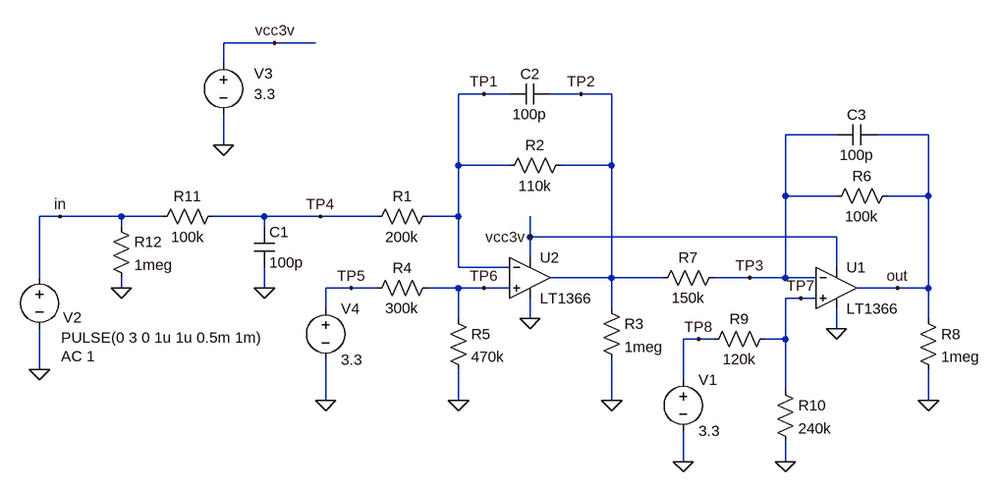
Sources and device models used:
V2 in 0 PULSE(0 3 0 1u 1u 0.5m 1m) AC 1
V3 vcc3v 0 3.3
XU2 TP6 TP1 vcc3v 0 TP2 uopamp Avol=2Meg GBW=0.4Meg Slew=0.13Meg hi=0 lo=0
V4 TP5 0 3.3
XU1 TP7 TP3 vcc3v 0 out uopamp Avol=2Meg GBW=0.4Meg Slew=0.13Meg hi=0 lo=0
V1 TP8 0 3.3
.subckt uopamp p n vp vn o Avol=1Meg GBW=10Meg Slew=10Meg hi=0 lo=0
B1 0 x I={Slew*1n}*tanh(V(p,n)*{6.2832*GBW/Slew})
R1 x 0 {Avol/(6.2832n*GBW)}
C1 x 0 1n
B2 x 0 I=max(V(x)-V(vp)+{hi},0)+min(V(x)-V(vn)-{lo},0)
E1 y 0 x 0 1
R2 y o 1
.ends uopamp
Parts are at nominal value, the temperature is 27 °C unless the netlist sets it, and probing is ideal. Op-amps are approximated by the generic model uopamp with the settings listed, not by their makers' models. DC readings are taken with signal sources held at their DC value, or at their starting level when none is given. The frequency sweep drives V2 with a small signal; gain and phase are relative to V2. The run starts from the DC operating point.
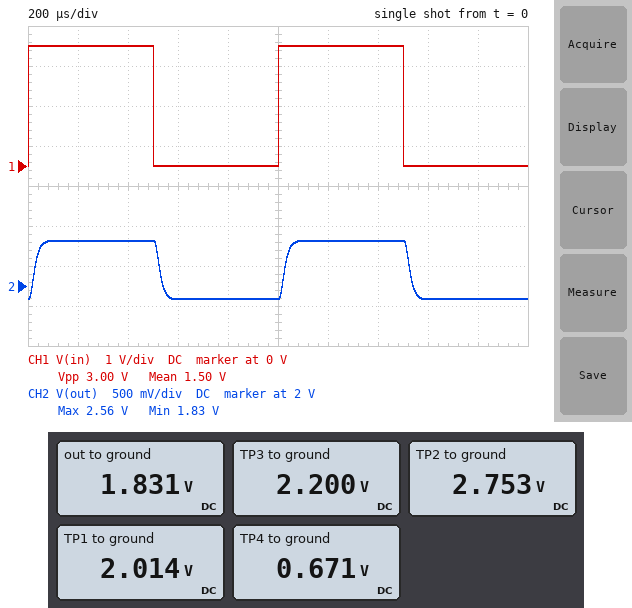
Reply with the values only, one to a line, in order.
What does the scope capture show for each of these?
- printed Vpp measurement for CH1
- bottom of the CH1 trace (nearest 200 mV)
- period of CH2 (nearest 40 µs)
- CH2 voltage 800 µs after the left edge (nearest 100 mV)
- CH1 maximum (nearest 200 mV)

3.00 V
0 V
1.00 ms
1.8 V
3.0 V
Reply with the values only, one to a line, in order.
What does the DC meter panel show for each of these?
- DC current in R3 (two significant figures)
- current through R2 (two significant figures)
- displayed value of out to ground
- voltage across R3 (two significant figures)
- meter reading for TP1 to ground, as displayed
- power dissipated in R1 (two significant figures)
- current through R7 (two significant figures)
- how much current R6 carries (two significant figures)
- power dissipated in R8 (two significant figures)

2.8 µA
6.7 µA
1.831 V
2.8 V
2.014 V
9.0 µW
3.7 µA
3.7 µA
3.4 µW
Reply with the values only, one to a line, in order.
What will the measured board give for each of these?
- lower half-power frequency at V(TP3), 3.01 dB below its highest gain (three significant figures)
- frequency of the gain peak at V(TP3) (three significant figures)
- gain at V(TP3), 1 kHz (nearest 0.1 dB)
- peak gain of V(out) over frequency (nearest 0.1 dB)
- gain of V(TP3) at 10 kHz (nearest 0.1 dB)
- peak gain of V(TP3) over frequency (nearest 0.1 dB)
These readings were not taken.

5.29 kHz
12.1 kHz
-64.3 dB
-12.2 dB
-48.2 dB
-48.0 dB
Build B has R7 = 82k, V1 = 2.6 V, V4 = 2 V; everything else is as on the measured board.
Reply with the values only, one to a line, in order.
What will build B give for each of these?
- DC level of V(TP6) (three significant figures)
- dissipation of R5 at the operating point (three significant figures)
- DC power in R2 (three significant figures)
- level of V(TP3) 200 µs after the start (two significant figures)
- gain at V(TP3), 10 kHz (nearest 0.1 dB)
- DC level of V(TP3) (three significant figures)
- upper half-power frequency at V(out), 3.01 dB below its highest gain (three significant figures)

1.22 V
3.17 µW
1.82 µW
1.7 V
-43.0 dB
1.73 V
8.48 kHz
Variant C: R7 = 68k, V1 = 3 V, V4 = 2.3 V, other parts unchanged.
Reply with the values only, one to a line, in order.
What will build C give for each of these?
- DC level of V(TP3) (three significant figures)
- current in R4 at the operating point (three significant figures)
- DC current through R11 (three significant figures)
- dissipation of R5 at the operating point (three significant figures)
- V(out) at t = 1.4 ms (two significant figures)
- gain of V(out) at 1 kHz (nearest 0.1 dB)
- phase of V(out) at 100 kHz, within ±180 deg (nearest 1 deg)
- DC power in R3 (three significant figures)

2.00 V
2.99 µA
4.68 µA
4.19 µW
3.3 V
-5.4 dB
93 deg
3.68 µW
